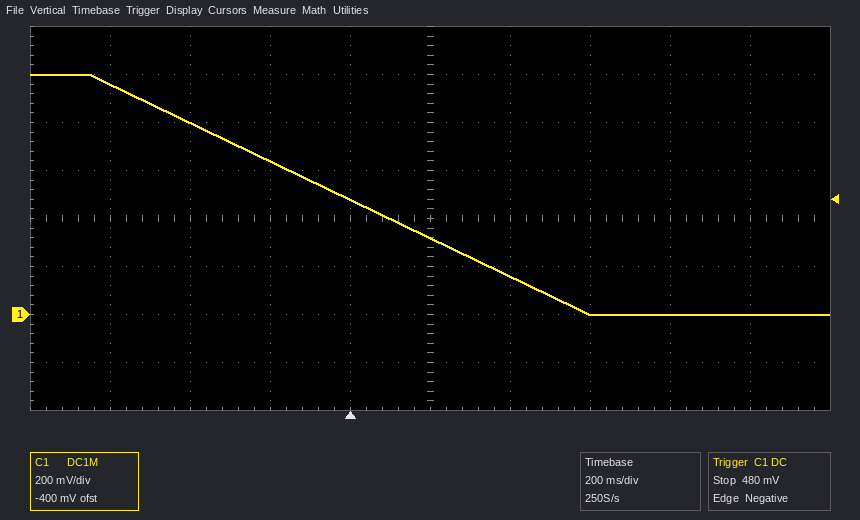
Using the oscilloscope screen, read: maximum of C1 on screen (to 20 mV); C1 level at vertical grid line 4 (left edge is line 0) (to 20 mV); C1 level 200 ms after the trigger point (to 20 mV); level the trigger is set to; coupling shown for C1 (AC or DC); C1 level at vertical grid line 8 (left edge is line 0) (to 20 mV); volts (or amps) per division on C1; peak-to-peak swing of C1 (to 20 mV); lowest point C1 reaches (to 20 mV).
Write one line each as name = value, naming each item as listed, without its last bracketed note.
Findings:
maximum of C1 on screen = 1.00 V
C1 level at vertical grid line 4 (left edge is line 0) = 480 mV
C1 level 200 ms after the trigger point = 320 mV
level the trigger is set to = 480 mV
coupling shown for C1 = DC
C1 level at vertical grid line 8 (left edge is line 0) = 0 mV
volts (or amps) per division on C1 = 200 mV
peak-to-peak swing of C1 = 1.00 V
lowest point C1 reaches = 0 mV
